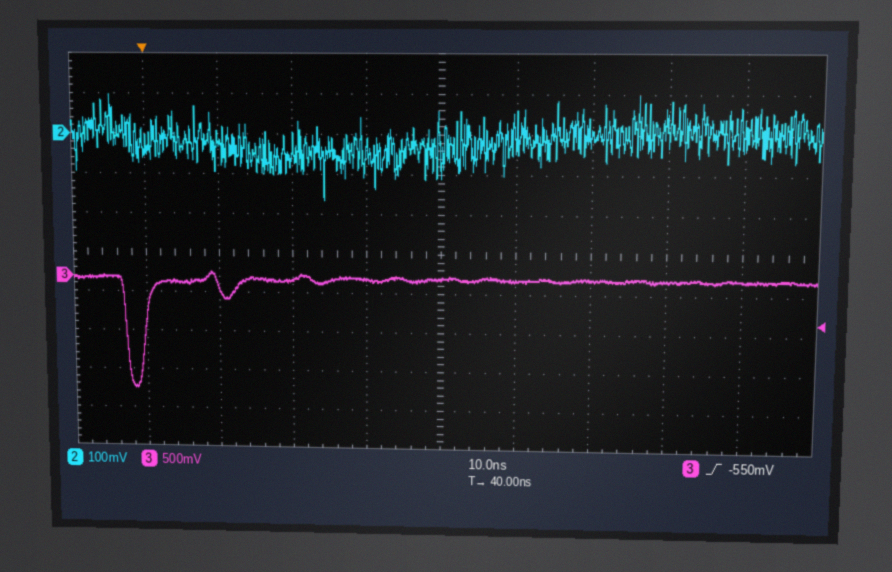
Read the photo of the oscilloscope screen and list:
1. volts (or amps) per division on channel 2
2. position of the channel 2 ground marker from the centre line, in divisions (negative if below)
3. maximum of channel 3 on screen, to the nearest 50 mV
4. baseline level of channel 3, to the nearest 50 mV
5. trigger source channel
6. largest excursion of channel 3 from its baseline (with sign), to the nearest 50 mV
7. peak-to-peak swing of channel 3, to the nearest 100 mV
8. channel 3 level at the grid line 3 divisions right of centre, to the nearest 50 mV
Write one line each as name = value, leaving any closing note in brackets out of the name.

volts (or amps) per division on channel 2 = 100 mV
position of the channel 2 ground marker from the centre line, in divisions = +3.0 div
maximum of channel 3 on screen, to the nearest 50 mV = 50 mV
baseline level of channel 3, to the nearest 50 mV = 0 mV
trigger source channel = channel 3
largest excursion of channel 3 from its baseline (with sign), to the nearest 50 mV = -1.40 V
peak-to-peak swing of channel 3, to the nearest 100 mV = 1.50 V
channel 3 level at the grid line 3 divisions right of centre, to the nearest 50 mV = 0 mV
